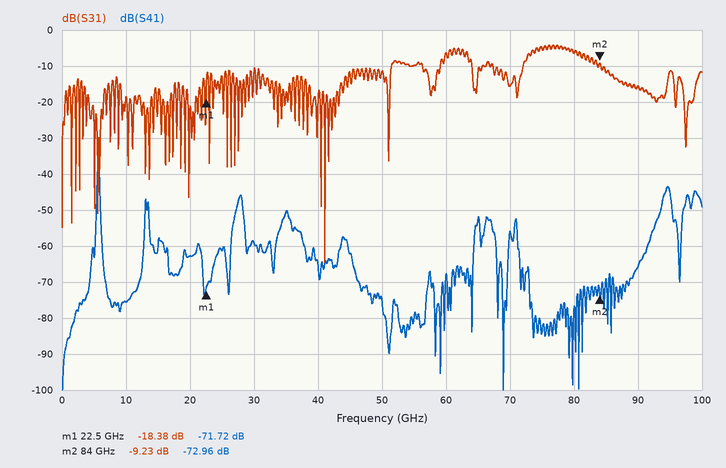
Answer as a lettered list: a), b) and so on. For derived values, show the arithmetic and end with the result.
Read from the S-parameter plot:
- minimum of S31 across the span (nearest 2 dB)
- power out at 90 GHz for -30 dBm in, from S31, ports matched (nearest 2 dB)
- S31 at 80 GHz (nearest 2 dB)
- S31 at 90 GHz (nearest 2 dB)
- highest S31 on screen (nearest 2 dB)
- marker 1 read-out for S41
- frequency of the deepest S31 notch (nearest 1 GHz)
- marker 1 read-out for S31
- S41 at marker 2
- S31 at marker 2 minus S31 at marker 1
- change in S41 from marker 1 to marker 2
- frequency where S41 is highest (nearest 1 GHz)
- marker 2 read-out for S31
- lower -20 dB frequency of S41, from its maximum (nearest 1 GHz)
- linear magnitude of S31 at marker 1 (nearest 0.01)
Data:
a) -64 dB
b) -30 dBm + (-16 dB) = -46 dBm
c) -6 dB
d) -16 dB
e) -4 dB
f) -71.72 dB
g) 41 GHz
h) -18.38 dB
i) -72.96 dB
j) -9.23 − (-18.38) = 9.15 dB
k) -72.96 − (-71.72) = -1.24 dB
l) 6 GHz
m) -9.23 dB
n) 5 GHz
o) 10^(-18.38/20) ≈ 0.12
